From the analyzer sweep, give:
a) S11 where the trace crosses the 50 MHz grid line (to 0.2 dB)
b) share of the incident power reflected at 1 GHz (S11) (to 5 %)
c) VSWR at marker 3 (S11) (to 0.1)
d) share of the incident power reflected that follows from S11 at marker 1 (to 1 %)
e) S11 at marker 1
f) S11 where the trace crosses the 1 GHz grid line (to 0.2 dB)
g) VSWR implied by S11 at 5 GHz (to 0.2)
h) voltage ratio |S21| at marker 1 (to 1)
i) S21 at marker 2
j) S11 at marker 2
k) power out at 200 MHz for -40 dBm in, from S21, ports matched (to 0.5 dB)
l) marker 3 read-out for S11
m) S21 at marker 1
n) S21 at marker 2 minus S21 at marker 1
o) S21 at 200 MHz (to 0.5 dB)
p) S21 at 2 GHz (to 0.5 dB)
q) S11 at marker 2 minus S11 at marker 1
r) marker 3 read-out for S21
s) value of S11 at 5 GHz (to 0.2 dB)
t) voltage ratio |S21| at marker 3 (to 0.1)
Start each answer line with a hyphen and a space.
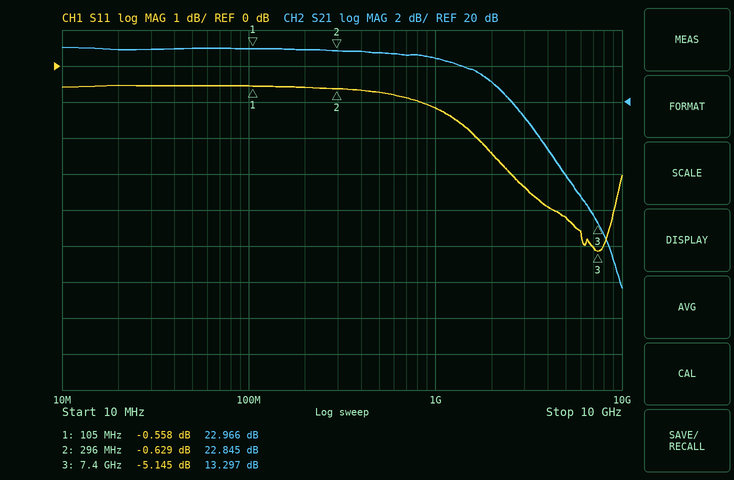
- -0.6 dB
- 75 %
- 3.5
- 88 %
- -0.558 dB
- -1.2 dB
- 4.2
- 14
- 22.845 dB
- -0.629 dB
- -17.0 dBm
- -5.145 dB
- 22.966 dB
- -0.121 dB
- 23.0 dB
- 21.0 dB
- -0.071 dB
- 13.297 dB
- -4.2 dB
- 4.6
